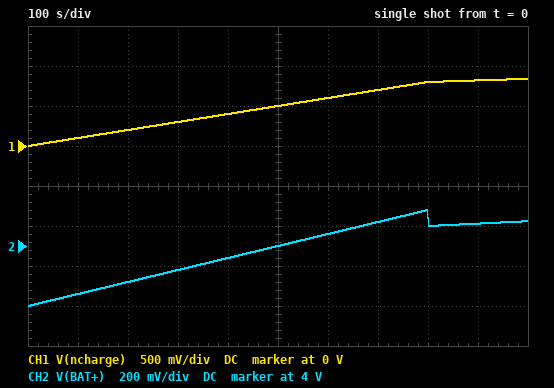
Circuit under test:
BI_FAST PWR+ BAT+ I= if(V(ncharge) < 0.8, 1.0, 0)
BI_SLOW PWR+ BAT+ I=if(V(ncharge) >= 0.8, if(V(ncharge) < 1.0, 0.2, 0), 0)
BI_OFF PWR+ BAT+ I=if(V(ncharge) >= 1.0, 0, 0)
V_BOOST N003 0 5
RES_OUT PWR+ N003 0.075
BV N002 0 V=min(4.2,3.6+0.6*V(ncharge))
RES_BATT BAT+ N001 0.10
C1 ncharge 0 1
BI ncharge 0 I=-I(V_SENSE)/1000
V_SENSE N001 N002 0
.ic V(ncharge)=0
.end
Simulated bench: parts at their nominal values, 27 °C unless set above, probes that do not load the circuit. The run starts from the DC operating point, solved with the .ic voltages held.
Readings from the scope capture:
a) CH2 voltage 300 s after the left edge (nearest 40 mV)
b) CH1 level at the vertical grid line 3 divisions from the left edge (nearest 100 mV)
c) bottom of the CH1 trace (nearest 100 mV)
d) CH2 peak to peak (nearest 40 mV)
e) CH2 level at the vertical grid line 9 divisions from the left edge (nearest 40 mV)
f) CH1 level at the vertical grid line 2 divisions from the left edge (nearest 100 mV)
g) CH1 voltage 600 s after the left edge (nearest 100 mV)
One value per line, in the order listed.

3.88 V
300 mV
0 V
480 mV
4.12 V
200 mV
600 mV
